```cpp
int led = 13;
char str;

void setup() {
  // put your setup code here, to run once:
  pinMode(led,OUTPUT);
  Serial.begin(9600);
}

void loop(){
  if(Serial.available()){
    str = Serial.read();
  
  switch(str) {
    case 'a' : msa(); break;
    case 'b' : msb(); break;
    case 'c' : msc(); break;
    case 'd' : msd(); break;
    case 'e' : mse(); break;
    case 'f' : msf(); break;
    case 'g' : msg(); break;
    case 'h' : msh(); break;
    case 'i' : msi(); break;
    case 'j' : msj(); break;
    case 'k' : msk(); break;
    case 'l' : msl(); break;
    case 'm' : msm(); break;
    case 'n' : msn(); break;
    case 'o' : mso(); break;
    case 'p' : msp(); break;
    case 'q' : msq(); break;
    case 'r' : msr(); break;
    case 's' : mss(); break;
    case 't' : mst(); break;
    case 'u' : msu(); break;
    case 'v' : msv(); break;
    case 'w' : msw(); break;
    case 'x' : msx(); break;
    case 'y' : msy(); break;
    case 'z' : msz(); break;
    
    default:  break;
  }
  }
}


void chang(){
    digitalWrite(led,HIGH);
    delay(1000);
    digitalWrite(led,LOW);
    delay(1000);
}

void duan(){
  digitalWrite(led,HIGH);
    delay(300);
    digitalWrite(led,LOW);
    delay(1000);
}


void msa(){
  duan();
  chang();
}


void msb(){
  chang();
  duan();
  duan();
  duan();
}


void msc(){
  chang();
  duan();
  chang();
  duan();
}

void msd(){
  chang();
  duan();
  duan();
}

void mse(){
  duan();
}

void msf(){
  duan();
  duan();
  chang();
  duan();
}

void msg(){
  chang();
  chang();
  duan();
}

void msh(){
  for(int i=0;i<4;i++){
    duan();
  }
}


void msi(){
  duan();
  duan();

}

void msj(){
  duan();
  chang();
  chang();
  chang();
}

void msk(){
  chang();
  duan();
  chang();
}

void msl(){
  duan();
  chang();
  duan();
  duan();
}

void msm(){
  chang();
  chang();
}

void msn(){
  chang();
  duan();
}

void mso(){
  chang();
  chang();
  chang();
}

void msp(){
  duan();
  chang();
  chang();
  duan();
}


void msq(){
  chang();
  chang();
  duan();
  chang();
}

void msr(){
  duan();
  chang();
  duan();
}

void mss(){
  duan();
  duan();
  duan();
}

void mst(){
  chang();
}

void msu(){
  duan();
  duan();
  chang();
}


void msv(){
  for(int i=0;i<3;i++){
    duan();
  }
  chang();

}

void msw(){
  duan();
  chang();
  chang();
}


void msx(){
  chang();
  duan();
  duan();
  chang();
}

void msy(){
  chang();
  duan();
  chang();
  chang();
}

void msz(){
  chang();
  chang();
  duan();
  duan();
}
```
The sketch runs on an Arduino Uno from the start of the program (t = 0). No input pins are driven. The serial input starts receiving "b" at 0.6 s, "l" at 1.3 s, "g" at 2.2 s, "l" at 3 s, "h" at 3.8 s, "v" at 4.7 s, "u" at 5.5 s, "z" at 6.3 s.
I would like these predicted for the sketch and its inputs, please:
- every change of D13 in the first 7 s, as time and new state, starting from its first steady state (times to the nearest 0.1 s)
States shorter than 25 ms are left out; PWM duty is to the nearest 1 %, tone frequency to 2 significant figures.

0 s low; 0.6 s high; 1.6 s low; 2.6 s high; 2.9 s low; 3.9 s high; 4.2 s low; 5.2 s high; 5.5 s low; 6.5 s high; 6.8 s low
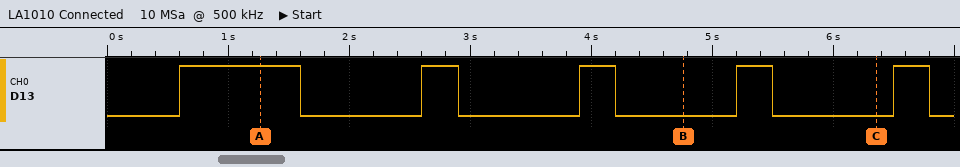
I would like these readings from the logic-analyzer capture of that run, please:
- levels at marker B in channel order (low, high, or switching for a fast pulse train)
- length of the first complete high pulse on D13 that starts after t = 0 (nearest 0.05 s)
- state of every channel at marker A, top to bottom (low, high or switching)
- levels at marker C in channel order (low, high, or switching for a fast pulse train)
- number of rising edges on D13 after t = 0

D13 low
1.00 s
D13 high
D13 low
5
